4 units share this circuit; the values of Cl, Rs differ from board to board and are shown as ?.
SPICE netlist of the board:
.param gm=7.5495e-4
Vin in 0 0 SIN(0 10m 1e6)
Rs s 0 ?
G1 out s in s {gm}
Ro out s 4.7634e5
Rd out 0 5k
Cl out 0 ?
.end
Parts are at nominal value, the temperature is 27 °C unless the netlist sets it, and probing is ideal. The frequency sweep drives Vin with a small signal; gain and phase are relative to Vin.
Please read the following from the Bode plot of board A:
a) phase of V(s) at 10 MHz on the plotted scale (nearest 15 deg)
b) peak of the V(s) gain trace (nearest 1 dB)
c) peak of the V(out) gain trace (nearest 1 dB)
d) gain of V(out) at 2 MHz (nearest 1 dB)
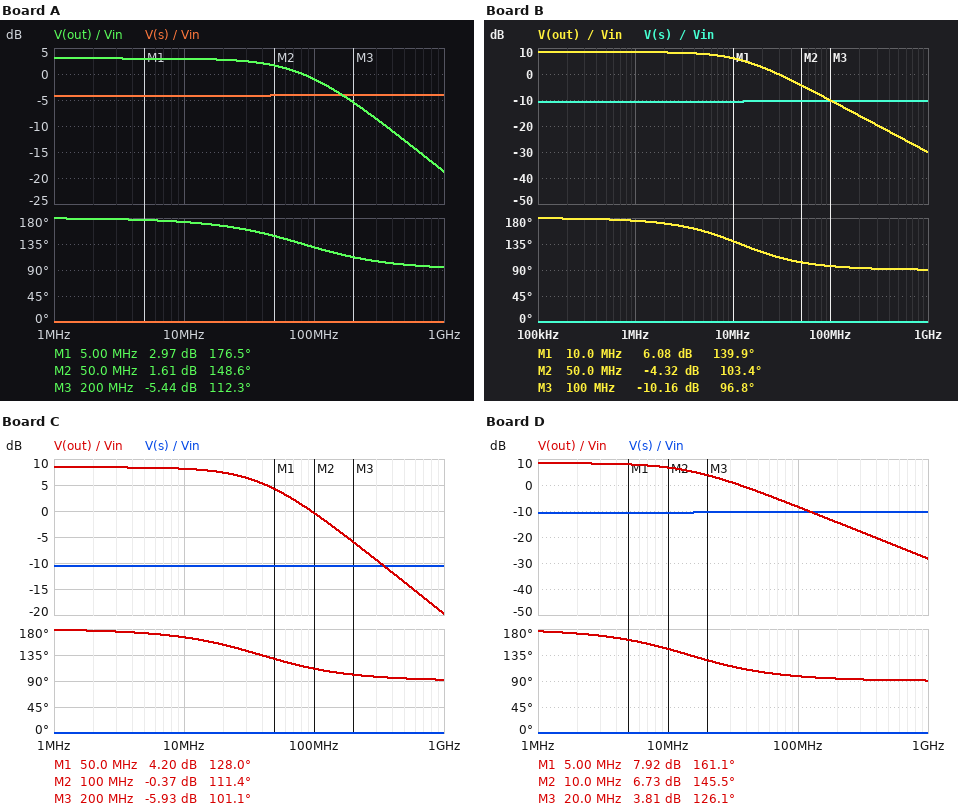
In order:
0 deg
-4 dB
3 dB
3 dB
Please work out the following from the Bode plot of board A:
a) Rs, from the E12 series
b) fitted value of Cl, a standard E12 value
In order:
2.2 kΩ
390 fF
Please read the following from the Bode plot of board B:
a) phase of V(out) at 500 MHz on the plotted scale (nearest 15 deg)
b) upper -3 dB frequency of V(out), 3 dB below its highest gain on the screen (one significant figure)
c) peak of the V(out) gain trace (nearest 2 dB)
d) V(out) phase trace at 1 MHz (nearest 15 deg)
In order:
90 deg
10 MHz
8 dB
180 deg
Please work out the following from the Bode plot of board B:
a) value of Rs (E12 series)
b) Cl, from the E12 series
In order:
560 Ω
2.7 pF
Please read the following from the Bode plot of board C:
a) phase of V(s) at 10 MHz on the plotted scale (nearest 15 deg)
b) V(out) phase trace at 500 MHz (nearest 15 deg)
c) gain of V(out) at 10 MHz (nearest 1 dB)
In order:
0 deg
90 deg
8 dB
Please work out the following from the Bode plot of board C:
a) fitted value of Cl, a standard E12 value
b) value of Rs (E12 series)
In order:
820 fF
560 Ω
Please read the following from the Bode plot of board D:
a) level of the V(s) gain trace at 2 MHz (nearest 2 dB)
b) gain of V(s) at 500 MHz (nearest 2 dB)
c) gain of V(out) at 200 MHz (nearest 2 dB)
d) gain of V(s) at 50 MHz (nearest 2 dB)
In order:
-10 dB
-10 dB
-14 dB
-10 dB
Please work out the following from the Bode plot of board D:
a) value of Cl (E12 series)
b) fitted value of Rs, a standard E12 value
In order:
2.2 pF
560 Ω
